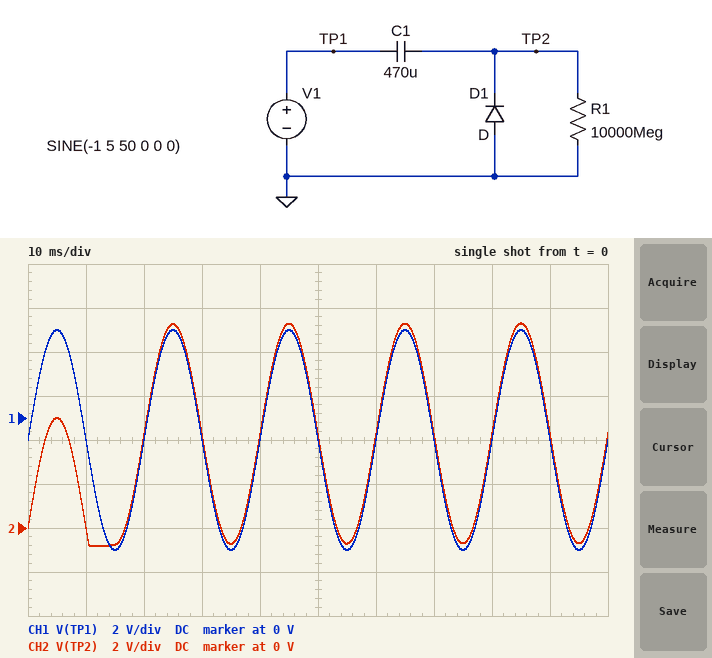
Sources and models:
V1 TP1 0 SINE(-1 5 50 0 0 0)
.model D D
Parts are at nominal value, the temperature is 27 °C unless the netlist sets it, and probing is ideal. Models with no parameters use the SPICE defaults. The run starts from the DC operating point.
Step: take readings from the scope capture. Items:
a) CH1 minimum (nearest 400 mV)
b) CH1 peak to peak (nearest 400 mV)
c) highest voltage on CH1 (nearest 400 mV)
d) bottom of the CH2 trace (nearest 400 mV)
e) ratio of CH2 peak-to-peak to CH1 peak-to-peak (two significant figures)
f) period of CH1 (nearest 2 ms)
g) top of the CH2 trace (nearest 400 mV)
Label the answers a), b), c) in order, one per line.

a) -6.0 V
b) 10.0 V
c) 4.0 V
d) -800 mV
e) 1.0
f) 20 ms
g) 9.2 V
